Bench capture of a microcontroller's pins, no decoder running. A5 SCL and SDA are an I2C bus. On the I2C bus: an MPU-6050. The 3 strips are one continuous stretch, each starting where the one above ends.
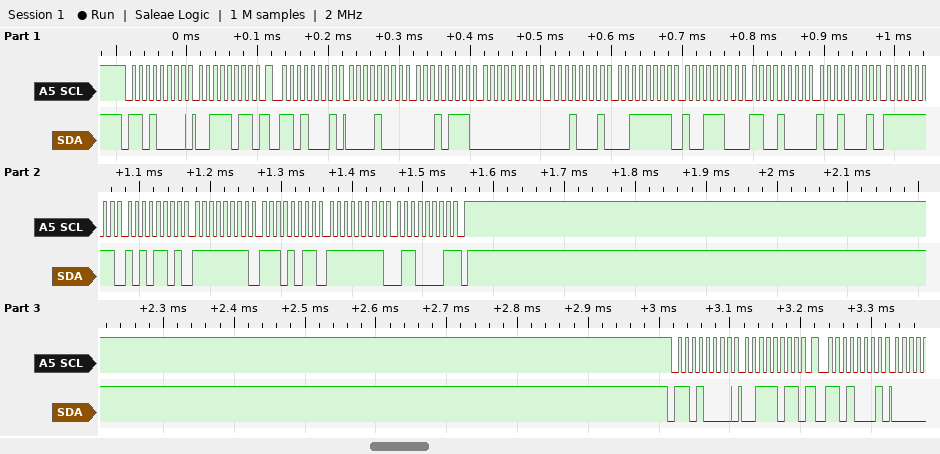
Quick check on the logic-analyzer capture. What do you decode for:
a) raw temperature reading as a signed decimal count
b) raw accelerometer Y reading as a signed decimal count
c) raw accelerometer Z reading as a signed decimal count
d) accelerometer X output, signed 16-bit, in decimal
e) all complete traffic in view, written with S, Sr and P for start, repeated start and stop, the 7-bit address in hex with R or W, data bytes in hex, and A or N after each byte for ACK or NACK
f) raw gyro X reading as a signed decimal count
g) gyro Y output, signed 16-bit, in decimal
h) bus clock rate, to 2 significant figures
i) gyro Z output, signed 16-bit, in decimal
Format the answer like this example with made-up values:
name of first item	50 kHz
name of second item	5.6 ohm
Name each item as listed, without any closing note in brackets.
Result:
raw temperature reading as a signed decimal count	-14191
raw accelerometer Y reading as a signed decimal count	17
raw accelerometer Z reading as a signed decimal count	16284
accelerometer X output, signed 16-bit, in decimal	2071
all complete traffic in view, written with S, Sr and P for start, repeated start and stop, the 7-bit address in hex with R or W, data bytes in hex, and A or N after each byte for ACK or NACK	S 68W A 3B A Sr 68R A 08 A 17 A 00 A 11 A 3F A 9C A C8 A 91 A FF A AD A FF A EB A FF A 61 N P S 68W A 3B A Sr 68R A
raw gyro X reading as a signed decimal count	-83
gyro Y output, signed 16-bit, in decimal	-21
bus clock rate, to 2 significant figures	100 kHz
gyro Z output, signed 16-bit, in decimal	-159
